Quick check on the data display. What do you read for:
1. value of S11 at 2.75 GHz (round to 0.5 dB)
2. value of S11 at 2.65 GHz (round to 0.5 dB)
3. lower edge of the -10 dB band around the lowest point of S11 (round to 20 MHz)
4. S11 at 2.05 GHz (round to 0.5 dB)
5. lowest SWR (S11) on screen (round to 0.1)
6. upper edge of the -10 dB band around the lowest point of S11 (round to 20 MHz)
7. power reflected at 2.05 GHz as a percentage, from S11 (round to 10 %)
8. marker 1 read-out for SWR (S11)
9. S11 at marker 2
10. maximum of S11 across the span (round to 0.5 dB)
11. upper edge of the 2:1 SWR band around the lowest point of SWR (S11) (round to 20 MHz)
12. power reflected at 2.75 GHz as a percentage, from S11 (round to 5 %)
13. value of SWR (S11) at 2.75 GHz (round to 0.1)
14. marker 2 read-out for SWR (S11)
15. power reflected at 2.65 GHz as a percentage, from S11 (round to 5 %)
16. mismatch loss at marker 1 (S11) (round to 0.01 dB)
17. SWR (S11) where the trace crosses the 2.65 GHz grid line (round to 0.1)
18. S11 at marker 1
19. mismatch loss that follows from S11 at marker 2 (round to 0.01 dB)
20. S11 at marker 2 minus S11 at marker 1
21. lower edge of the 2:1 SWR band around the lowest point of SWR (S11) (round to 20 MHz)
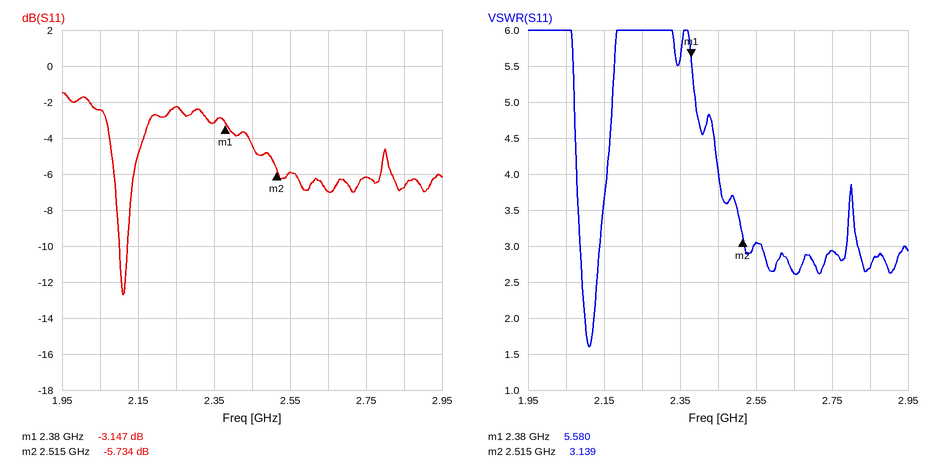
-6.0 dB
-7.0 dB
2.10 GHz
-2.5 dB
1.6
2.12 GHz
60 %
5.580
-5.734 dB
-1.5 dB
2.12 GHz
25 %
2.9
3.139
20 %
2.88 dB
2.6
-3.147 dB
1.35 dB
-2.587 dB
2.10 GHz
